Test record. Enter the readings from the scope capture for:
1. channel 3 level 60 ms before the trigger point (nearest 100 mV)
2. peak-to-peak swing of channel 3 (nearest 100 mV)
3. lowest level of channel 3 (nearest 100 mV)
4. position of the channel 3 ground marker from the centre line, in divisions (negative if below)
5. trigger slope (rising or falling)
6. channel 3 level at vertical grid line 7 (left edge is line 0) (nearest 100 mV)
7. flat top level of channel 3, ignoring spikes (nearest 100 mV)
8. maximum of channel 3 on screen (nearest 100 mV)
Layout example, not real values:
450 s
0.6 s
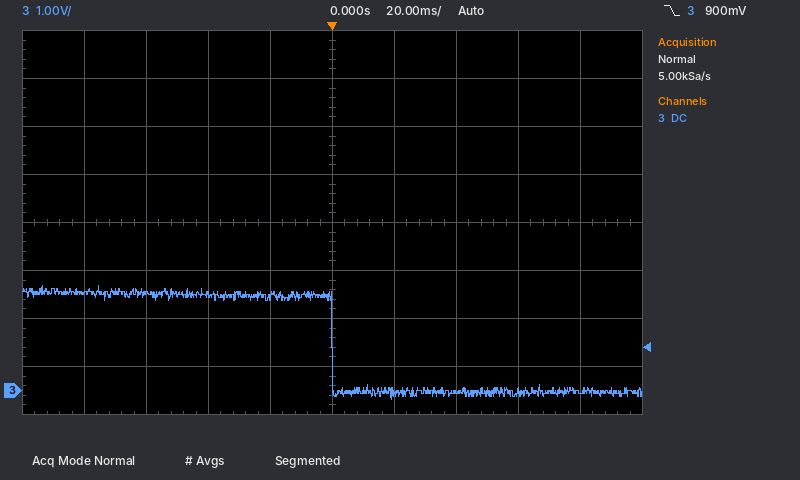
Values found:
2.0 V
2.4 V
-200 mV
-3.5 div
falling
0.0 V
2.0 V
2.2 V
